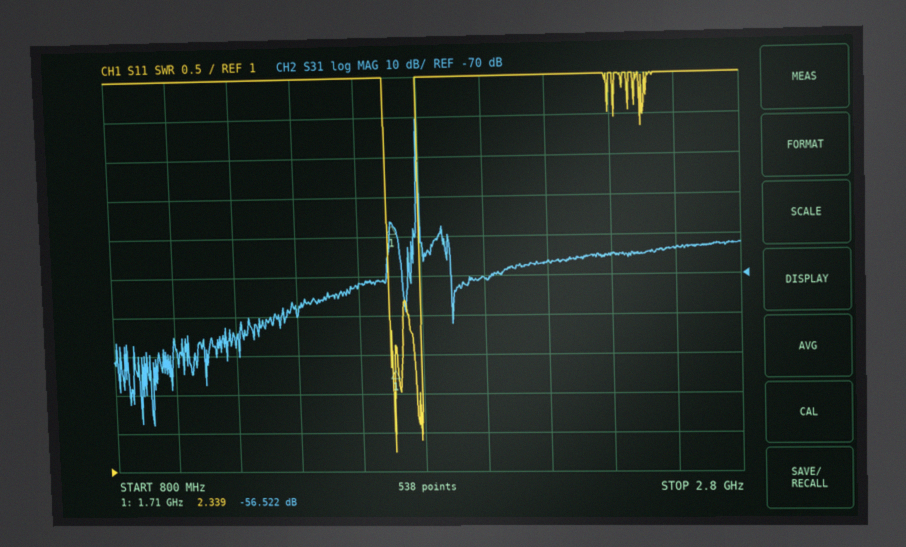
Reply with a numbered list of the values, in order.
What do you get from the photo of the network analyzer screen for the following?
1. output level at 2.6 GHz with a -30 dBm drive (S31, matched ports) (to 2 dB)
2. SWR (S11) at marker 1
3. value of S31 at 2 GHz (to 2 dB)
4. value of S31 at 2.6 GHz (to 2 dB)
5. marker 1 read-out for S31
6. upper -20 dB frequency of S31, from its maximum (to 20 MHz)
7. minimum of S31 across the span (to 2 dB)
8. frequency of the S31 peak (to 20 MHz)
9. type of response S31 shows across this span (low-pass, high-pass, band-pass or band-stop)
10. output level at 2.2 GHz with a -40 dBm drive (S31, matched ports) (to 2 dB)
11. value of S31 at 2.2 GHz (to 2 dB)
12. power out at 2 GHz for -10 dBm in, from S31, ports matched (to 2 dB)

1. -94 dBm
2. 2.339
3. -70 dB
4. -64 dB
5. -56.522 dB
6. 1.80 GHz
7. -108 dB
8. 1.80 GHz
9. band-pass
10. -106 dBm
11. -66 dB
12. -80 dBm
